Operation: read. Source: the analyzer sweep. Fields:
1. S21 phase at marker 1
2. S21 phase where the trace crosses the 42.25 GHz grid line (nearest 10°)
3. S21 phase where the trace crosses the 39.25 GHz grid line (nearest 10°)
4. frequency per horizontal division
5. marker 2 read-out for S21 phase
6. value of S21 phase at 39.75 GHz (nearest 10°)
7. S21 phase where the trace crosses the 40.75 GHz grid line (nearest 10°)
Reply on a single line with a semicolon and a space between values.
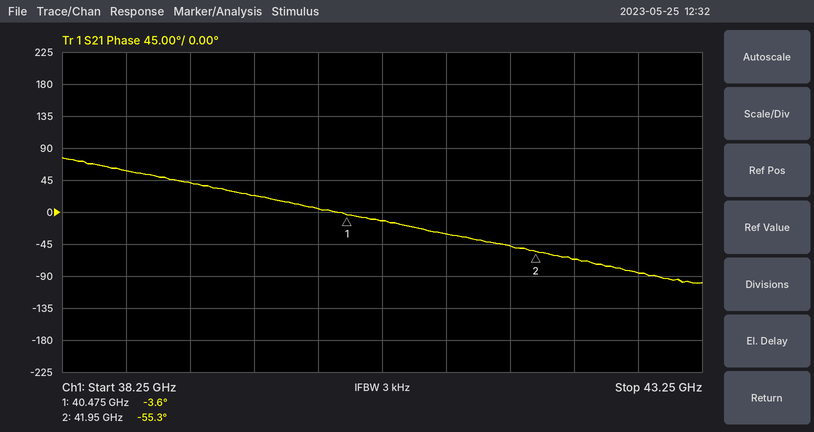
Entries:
-3.6°; -70°; 40°; 500 MHz; -55.3°; 20°; -10°
